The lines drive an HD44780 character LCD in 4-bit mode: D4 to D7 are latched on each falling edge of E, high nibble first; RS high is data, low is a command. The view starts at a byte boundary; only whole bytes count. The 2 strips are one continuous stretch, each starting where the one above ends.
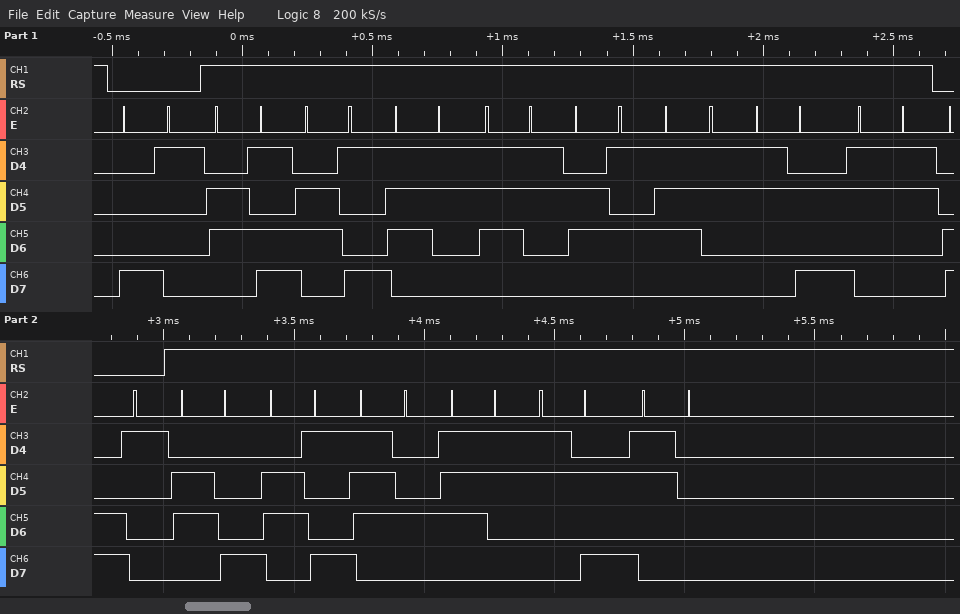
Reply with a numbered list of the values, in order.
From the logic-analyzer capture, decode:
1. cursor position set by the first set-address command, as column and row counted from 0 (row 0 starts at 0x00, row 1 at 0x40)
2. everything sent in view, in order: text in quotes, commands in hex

1. column 1, row 0
2. 0x81 "misses:3" 0xC1 "hits:0"
